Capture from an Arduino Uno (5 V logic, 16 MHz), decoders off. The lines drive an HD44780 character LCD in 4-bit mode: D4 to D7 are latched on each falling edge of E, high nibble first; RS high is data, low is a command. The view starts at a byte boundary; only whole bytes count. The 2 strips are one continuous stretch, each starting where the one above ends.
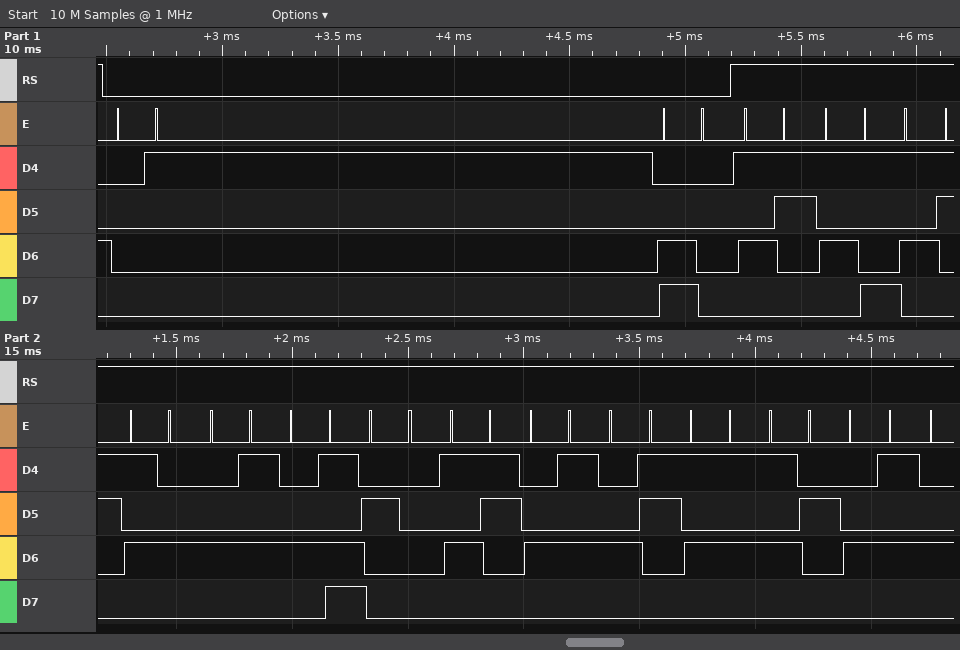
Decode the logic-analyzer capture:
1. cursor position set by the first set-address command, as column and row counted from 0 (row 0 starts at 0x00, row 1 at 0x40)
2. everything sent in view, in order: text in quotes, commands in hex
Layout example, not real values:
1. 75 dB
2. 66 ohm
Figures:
1. column 0, row 1
2. 0x01 0xC0 "SYSTEM SECURE"
